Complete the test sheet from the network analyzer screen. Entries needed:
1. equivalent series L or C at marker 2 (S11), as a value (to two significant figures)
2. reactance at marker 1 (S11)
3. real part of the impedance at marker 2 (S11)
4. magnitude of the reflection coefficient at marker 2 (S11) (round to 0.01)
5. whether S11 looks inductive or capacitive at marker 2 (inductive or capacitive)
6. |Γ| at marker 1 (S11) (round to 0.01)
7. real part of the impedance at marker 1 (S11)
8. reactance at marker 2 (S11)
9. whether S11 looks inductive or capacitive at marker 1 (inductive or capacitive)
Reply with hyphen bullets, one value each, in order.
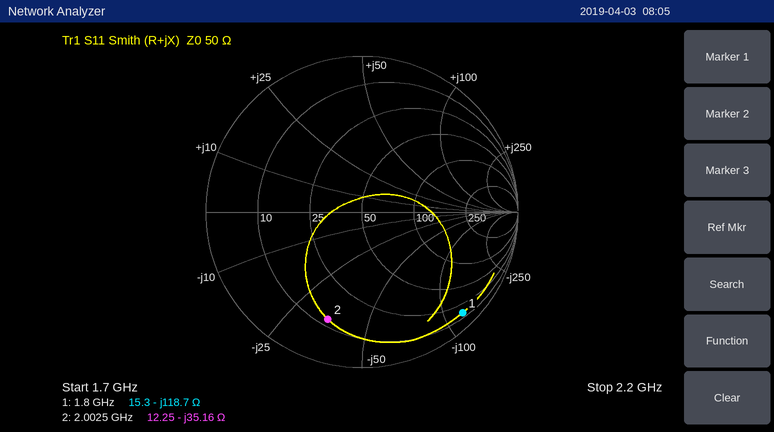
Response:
- 2.3 pF
- -118.7 Ω
- 12.25 Ω
- 0.72
- capacitive
- 0.91
- 15.3 Ω
- -35.16 Ω
- capacitive
